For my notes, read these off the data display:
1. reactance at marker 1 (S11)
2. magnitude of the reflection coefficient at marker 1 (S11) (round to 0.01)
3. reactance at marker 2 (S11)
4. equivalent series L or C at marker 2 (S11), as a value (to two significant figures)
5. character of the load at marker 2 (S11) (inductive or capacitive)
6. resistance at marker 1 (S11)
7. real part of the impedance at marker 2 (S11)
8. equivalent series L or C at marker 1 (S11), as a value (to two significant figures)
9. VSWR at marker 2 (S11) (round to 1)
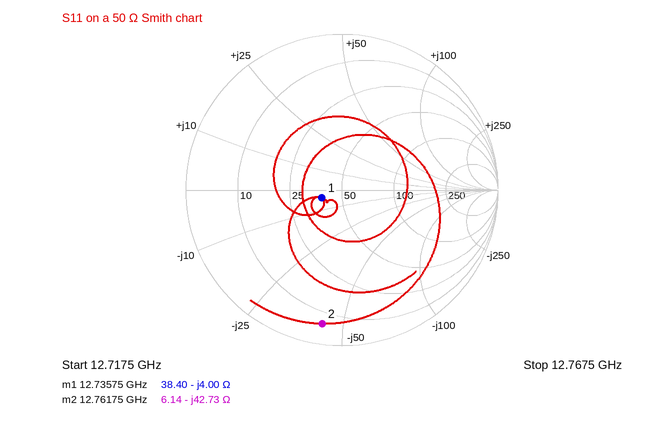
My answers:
-4.00 Ω
0.14
-42.73 Ω
290 fF
capacitive
38.40 Ω
6.14 Ω
3.1 pF
14
